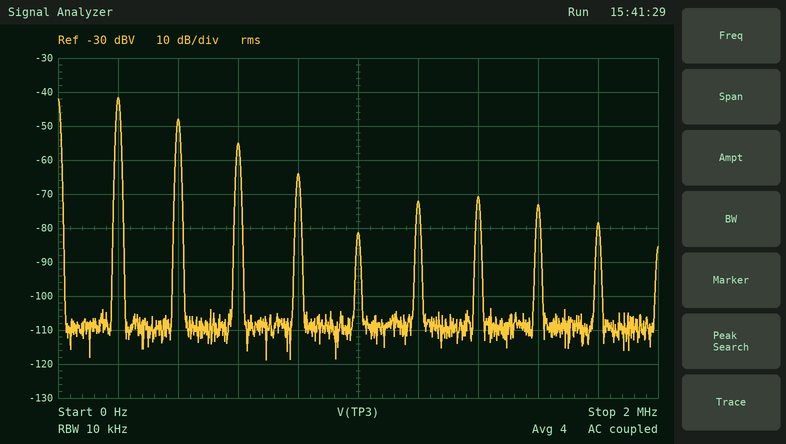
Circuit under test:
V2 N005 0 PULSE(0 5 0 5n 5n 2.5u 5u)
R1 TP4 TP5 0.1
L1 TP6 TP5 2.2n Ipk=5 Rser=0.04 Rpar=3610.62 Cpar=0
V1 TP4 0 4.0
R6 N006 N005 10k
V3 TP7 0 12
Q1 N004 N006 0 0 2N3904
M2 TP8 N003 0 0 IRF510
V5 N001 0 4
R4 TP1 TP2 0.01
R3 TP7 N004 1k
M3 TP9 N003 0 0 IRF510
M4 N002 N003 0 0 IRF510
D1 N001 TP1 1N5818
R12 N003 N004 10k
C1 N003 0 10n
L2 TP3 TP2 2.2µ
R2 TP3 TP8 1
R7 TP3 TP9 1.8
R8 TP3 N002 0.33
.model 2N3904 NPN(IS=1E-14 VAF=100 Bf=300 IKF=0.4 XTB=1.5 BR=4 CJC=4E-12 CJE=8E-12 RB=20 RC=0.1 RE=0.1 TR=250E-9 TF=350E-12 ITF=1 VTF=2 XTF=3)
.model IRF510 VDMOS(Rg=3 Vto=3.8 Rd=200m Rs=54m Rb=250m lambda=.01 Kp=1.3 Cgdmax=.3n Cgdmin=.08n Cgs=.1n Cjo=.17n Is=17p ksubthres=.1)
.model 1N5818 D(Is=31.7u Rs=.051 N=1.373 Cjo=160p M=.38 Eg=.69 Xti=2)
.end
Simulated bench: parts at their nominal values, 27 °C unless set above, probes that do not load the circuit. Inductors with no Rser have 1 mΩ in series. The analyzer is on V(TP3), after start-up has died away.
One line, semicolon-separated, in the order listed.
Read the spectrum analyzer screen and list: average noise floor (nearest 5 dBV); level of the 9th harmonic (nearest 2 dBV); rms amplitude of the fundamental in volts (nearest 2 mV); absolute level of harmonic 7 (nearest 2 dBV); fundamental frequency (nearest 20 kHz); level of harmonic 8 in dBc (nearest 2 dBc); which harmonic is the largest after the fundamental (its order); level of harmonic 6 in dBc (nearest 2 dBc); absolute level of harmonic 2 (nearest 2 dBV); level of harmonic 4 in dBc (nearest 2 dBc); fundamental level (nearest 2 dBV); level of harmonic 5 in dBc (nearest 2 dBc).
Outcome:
-110 dBV; -78 dBV; 8 mV; -70 dBV; 200 kHz; -32 dBc; 2; -30 dBc; -48 dBV; -22 dBc; -42 dBV; -40 dBc
